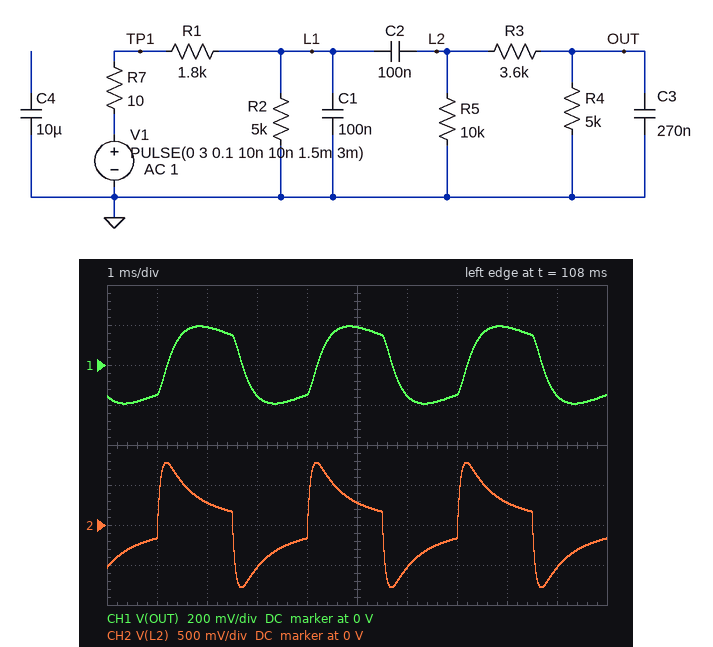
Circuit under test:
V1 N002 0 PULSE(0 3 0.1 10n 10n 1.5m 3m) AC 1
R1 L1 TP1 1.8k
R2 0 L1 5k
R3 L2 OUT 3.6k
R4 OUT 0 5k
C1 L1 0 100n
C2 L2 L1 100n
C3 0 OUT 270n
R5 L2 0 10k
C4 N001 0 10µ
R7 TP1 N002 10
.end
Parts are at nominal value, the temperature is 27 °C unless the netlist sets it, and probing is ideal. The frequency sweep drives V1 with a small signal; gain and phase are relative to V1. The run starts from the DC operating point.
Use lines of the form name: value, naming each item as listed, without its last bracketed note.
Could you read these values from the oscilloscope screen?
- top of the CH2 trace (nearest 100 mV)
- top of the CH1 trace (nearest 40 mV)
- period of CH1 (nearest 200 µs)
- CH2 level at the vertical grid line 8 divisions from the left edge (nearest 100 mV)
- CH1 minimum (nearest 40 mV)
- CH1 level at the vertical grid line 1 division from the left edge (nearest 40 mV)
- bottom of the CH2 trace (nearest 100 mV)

top of the CH2 trace: 800 mV
top of the CH1 trace: 200 mV
period of CH1: 3.0 ms
CH2 level at the vertical grid line 8 divisions from the left edge: 300 mV
CH1 minimum: -200 mV
CH1 level at the vertical grid line 1 division from the left edge: -160 mV
bottom of the CH2 trace: -800 mV
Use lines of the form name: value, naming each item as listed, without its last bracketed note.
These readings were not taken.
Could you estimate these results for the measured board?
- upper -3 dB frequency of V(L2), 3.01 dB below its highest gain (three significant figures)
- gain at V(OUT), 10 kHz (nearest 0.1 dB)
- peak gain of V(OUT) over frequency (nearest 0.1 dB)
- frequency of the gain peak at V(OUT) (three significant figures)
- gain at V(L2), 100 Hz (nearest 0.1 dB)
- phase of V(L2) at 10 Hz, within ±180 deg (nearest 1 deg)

upper -3 dB frequency of V(L2), 3.01 dB below its highest gain: 2.73 kHz
gain at V(OUT), 10 kHz: -57.0 dB
peak gain of V(OUT) over frequency: -18.4 dB
frequency of the gain peak at V(OUT): 230 Hz
gain at V(L2), 100 Hz: -15.3 dB
phase of V(L2) at 10 Hz, within ±180 deg: 86 deg
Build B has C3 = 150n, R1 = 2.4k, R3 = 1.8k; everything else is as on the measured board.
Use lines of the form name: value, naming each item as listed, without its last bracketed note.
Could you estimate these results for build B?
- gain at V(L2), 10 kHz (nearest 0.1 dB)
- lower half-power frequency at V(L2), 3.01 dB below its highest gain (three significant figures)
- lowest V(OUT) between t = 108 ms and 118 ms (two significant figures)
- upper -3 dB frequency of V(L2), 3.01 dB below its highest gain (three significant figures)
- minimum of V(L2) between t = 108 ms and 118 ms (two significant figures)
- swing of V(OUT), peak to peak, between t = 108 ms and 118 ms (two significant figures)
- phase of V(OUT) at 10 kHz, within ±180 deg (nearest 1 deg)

gain at V(L2), 10 kHz: -24.0 dB
lower half-power frequency at V(L2), 3.01 dB below its highest gain: 128 Hz
lowest V(OUT) between t = 108 ms and 118 ms: -300 mV
upper -3 dB frequency of V(L2), 3.01 dB below its highest gain: 2.32 kHz
minimum of V(L2) between t = 108 ms and 118 ms: -490 mV
swing of V(OUT), peak to peak, between t = 108 ms and 118 ms: 600 mV
phase of V(OUT) at 10 kHz, within ±180 deg: -158 deg
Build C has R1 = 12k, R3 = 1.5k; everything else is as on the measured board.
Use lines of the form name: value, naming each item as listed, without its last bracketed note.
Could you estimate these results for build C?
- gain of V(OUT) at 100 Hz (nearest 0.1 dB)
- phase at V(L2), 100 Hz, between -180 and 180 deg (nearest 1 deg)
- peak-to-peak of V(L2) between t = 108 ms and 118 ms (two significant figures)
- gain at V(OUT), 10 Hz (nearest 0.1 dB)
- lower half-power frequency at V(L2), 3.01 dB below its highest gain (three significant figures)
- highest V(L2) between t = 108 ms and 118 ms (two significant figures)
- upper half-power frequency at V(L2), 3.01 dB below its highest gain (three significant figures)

gain of V(OUT) at 100 Hz: -28.1 dB
phase at V(L2), 100 Hz, between -180 and 180 deg: 38 deg
peak-to-peak of V(L2) between t = 108 ms and 118 ms: 190 mV
gain at V(OUT), 10 Hz: -45.1 dB
lower half-power frequency at V(L2), 3.01 dB below its highest gain: 73.7 Hz
highest V(L2) between t = 108 ms and 118 ms: 94 mV
upper half-power frequency at V(L2), 3.01 dB below its highest gain: 1.11 kHz
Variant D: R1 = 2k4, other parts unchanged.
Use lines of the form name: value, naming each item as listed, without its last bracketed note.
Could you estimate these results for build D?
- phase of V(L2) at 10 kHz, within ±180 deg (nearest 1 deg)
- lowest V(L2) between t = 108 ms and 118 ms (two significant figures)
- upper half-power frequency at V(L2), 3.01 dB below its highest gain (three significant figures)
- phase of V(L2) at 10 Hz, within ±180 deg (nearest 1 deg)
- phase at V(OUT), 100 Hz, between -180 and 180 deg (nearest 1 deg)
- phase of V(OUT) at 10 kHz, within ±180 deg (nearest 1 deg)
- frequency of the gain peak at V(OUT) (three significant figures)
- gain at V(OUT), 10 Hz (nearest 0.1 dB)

phase of V(L2) at 10 kHz, within ±180 deg: -78 deg
lowest V(L2) between t = 108 ms and 118 ms: -630 mV
upper half-power frequency at V(L2), 3.01 dB below its highest gain: 2.46 kHz
phase of V(L2) at 10 Hz, within ±180 deg: 86 deg
phase at V(OUT), 100 Hz, between -180 and 180 deg: 34 deg
phase of V(OUT) at 10 kHz, within ±180 deg: -166 deg
frequency of the gain peak at V(OUT): 217 Hz
gain at V(OUT), 10 Hz: -38.9 dB
